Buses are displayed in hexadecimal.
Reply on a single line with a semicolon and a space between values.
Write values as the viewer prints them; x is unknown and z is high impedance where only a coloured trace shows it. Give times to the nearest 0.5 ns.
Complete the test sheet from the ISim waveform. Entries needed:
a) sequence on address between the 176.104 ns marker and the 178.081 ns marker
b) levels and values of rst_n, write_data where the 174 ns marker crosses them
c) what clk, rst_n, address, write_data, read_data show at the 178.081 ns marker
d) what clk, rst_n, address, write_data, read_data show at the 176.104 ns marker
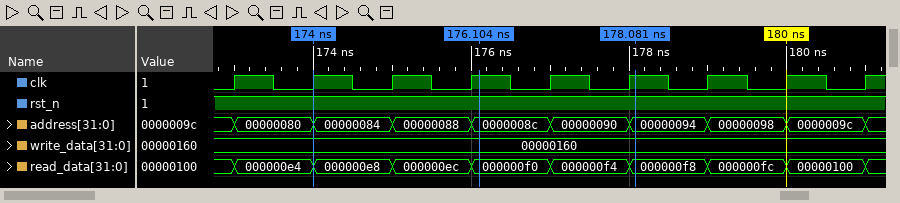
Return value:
0000008c, 00000090, 00000094; rst_n=1, write_data=00000160; clk=1, rst_n=1, address=00000094, write_data=00000160, read_data=000000f8; clk=1, rst_n=1, address=0000008c, write_data=00000160, read_data=000000f0
